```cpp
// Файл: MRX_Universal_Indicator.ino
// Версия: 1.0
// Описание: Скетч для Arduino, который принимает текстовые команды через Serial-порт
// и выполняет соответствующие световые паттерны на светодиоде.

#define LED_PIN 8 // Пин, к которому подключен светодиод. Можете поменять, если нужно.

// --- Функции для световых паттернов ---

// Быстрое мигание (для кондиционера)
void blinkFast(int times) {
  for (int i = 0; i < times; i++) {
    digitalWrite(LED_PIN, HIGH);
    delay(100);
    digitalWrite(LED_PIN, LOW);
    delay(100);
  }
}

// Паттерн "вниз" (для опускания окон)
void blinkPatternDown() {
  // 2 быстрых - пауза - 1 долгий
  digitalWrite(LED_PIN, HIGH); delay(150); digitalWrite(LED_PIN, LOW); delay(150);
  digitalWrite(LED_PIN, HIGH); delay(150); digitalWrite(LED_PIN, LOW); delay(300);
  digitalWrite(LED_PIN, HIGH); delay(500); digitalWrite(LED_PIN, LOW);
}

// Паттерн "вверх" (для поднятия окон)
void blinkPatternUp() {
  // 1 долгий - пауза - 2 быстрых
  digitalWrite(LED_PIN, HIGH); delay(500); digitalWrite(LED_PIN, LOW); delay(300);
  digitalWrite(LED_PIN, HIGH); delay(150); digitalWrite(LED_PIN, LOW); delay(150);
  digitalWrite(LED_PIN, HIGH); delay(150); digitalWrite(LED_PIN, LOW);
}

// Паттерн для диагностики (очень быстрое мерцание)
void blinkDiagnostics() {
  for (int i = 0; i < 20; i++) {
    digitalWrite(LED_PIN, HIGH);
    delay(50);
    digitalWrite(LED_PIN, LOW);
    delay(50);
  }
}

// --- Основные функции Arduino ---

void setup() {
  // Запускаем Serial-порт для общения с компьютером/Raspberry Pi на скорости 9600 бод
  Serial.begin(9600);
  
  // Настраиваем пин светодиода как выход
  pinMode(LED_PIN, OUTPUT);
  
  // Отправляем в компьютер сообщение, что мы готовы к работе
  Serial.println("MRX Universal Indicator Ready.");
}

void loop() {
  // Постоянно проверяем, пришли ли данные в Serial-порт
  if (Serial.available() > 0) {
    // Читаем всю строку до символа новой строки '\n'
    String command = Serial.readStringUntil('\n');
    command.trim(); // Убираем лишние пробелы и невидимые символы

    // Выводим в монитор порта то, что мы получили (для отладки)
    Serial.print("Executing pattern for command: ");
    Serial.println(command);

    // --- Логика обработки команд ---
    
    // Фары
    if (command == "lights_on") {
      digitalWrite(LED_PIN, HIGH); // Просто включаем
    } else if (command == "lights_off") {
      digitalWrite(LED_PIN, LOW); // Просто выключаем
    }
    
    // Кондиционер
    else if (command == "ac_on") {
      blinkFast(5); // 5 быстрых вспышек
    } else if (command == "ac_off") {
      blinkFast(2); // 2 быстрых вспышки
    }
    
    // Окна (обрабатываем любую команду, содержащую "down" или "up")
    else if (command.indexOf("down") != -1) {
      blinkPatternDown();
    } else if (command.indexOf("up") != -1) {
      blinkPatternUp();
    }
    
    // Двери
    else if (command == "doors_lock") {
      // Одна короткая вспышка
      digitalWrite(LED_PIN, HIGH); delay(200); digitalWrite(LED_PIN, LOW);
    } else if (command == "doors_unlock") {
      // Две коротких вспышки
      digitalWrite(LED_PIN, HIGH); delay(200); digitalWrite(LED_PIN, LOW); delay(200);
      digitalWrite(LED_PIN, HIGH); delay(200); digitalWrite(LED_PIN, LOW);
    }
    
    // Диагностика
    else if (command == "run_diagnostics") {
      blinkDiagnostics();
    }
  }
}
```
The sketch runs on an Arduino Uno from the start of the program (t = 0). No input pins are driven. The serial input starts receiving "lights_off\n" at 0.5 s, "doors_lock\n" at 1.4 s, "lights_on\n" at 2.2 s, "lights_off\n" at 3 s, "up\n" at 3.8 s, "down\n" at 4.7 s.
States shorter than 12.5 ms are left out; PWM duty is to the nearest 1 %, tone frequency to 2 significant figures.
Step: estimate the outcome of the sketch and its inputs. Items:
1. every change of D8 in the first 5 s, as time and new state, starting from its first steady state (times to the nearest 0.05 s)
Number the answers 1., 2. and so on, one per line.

1. 0 s low; 1.4 s high; 1.6 s low; 2.2 s high; 3 s low; 3.8 s high; 4.3 s low; 4.6 s high; 4.75 s low; 4.9 s high
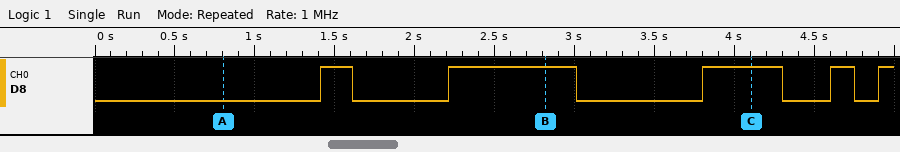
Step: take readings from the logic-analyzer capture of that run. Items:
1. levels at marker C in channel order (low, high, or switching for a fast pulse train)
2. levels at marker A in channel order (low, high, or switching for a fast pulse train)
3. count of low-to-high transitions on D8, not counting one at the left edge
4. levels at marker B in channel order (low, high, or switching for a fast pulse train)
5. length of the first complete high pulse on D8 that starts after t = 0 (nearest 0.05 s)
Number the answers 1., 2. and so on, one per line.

1. D8 high
2. D8 low
3. 5
4. D8 high
5. 0.20 s
